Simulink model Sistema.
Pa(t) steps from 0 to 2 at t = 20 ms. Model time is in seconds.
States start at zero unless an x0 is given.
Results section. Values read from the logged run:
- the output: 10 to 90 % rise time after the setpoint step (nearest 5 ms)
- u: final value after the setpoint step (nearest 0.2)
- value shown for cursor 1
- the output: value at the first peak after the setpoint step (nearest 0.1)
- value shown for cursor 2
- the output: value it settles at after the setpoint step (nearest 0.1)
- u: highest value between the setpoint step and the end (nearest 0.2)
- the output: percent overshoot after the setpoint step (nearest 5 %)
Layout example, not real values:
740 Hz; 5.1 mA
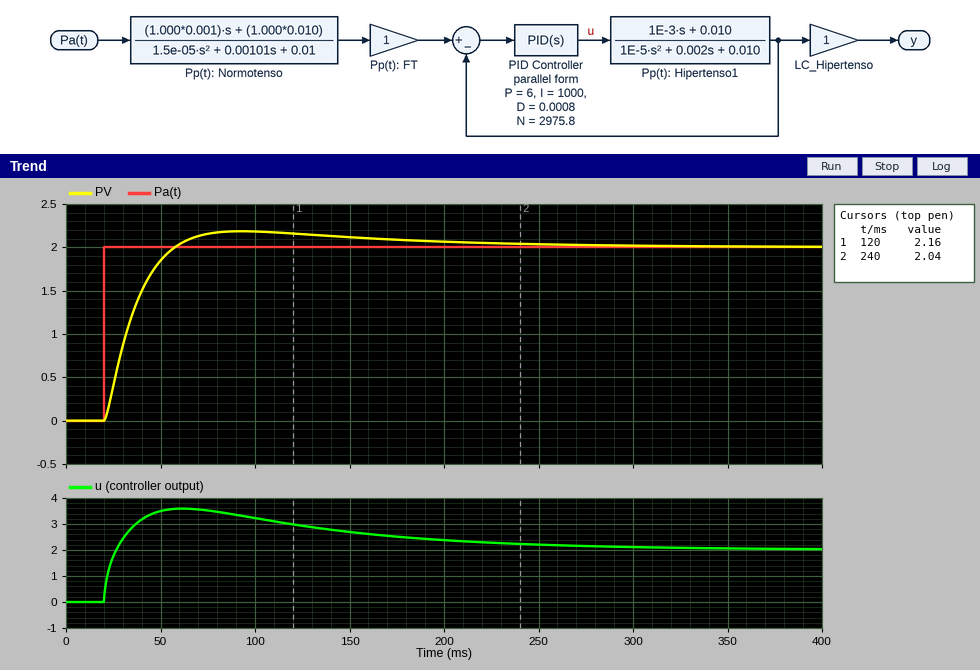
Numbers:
25 ms; 2.0; 2.16; 2.2; 2.04; 2.0; 3.6; 10 %
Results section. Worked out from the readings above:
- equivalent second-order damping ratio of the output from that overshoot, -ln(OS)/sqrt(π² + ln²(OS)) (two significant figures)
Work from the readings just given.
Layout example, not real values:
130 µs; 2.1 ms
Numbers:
0.59
